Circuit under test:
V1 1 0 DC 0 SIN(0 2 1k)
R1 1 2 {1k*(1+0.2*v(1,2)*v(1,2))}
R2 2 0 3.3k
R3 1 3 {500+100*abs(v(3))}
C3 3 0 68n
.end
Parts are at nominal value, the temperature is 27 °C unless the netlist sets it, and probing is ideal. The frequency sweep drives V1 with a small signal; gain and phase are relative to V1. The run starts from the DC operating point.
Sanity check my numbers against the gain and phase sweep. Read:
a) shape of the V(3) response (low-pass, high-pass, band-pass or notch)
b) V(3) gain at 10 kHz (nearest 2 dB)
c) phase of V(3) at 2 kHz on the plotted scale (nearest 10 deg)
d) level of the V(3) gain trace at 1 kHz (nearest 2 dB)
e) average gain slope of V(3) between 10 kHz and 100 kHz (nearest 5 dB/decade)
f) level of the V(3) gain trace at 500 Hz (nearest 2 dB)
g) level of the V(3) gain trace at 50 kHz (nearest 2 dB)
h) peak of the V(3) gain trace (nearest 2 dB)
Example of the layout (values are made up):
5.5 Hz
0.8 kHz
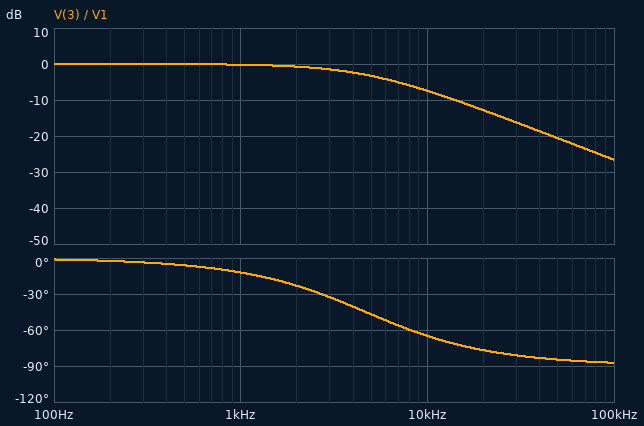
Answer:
low-pass
-8 dB
-20 deg
0 dB
-20 dB/decade
0 dB
-20 dB
0 dB
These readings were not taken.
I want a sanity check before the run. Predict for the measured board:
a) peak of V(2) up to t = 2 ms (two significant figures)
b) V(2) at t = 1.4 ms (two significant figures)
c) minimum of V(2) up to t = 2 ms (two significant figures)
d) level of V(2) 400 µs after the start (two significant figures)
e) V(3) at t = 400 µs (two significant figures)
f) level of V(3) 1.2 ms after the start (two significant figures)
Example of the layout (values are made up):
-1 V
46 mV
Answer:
1.5 V
900 mV
-1.5 V
900 mV
1.5 V
1.6 V
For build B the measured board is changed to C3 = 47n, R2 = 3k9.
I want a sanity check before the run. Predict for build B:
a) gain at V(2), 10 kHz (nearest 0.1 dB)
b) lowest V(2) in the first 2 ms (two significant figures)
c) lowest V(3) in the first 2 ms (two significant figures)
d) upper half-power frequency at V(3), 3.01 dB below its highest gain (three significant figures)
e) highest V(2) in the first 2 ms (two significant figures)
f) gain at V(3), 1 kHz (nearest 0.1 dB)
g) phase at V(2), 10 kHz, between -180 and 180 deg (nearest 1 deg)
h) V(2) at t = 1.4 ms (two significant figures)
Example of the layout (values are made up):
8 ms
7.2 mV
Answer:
-2.0 dB
-1.6 V
-2.0 V
6.77 kHz
1.6 V
-0.1 dB
0 deg
930 mV
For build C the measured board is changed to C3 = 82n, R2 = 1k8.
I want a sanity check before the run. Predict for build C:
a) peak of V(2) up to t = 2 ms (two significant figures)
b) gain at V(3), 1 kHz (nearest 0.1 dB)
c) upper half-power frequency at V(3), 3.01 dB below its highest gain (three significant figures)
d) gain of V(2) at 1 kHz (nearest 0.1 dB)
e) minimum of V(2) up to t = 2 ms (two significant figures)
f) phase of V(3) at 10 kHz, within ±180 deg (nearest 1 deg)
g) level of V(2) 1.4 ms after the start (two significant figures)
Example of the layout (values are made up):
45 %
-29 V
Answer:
1.2 V
-0.3 dB
3.88 kHz
-3.8 dB
-1.2 V
-69 deg
750 mV
